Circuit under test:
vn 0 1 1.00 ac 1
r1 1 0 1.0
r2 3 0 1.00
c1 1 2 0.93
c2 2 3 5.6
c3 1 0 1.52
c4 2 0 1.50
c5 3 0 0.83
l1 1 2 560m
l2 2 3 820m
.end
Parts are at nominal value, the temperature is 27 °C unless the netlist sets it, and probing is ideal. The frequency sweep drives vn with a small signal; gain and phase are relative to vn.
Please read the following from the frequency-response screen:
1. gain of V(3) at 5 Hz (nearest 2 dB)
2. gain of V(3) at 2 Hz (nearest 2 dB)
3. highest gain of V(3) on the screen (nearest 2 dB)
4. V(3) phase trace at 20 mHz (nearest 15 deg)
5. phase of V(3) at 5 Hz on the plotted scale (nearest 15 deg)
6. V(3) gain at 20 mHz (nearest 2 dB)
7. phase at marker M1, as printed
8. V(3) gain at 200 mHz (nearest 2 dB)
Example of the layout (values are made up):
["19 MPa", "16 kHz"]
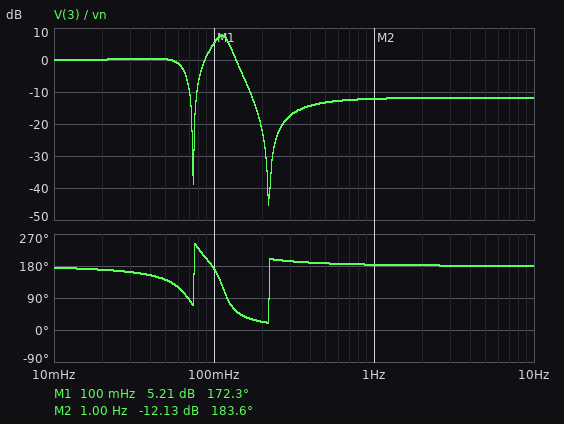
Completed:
["-12 dB", "-12 dB", "8 dB", "165 deg", "180 deg", "0 dB", "172.3 deg", "-22 dB"]
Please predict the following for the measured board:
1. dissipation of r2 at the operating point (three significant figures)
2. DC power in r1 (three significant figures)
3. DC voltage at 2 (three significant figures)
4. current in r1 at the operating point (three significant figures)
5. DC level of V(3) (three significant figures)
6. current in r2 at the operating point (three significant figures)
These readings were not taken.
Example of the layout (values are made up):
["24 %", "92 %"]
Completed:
["1.00 W", "1.00 W", "-1.00 V", "1.00 A", "-1.00 V", "1.00 A"]
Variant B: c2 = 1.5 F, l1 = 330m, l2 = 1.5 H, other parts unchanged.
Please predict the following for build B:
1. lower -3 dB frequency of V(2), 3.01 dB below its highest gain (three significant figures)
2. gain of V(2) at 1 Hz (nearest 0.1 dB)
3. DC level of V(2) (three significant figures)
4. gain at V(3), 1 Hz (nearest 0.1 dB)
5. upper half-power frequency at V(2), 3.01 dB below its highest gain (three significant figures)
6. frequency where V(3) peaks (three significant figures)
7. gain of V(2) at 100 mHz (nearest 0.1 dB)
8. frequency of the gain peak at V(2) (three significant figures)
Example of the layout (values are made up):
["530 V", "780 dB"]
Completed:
["155 mHz", "-10.6 dB", "-1.00 V", "-14.5 dB", "165 mHz", "161 mHz", "1.9 dB", "160 mHz"]
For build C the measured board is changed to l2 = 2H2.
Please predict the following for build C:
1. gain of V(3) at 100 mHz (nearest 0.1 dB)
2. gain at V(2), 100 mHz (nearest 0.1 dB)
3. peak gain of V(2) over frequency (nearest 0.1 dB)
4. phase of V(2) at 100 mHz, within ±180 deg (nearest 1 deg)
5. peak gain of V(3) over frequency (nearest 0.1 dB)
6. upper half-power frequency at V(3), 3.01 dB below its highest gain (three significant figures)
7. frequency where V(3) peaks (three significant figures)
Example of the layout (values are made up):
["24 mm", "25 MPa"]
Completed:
["5.7 dB", "7.6 dB", "8.7 dB", "136 deg", "7.0 dB", "126 mHz", "111 mHz"]
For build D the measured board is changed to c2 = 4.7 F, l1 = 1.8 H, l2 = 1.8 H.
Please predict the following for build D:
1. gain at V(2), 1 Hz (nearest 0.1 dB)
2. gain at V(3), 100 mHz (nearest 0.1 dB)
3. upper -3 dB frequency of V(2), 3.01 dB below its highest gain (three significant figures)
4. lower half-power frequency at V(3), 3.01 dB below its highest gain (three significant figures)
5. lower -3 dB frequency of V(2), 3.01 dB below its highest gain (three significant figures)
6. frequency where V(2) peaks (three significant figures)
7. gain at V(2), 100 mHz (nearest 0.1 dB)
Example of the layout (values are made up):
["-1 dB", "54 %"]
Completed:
["-10.7 dB", "-15.9 dB", "65.6 mHz", "61.9 mHz", "61.2 mHz", "63.4 mHz", "-13.3 dB"]
